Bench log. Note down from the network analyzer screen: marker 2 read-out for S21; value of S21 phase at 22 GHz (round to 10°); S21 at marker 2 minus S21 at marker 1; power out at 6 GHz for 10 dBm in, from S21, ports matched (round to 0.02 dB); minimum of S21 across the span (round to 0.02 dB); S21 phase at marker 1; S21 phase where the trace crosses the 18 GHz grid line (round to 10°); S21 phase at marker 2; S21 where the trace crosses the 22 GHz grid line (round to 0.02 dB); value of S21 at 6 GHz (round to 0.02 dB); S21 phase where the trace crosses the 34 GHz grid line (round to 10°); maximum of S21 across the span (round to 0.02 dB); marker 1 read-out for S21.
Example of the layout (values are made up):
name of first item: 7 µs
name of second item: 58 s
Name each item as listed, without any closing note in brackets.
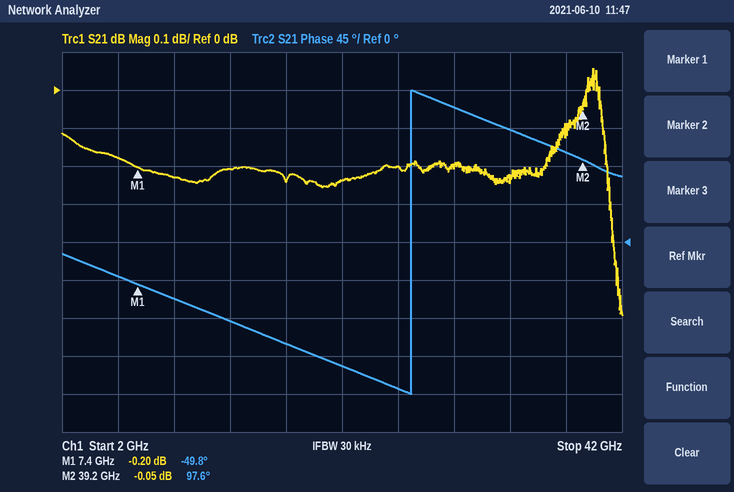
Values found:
marker 2 read-out for S21: -0.05 dB
value of S21 phase at 22 GHz: -150°
S21 at marker 2 minus S21 at marker 1: 0.15 dB
power out at 6 GHz for 10 dBm in, from S21, ports matched: 9.82 dBm
minimum of S21 across the span: -0.60 dB
S21 phase at marker 1: -49.8°
S21 phase where the trace crosses the 18 GHz grid line: -120°
S21 phase at marker 2: 97.6°
S21 where the trace crosses the 22 GHz grid line: -0.24 dB
value of S21 at 6 GHz: -0.18 dB
S21 phase where the trace crosses the 34 GHz grid line: 130°
maximum of S21 across the span: 0.06 dB
marker 1 read-out for S21: -0.20 dB
